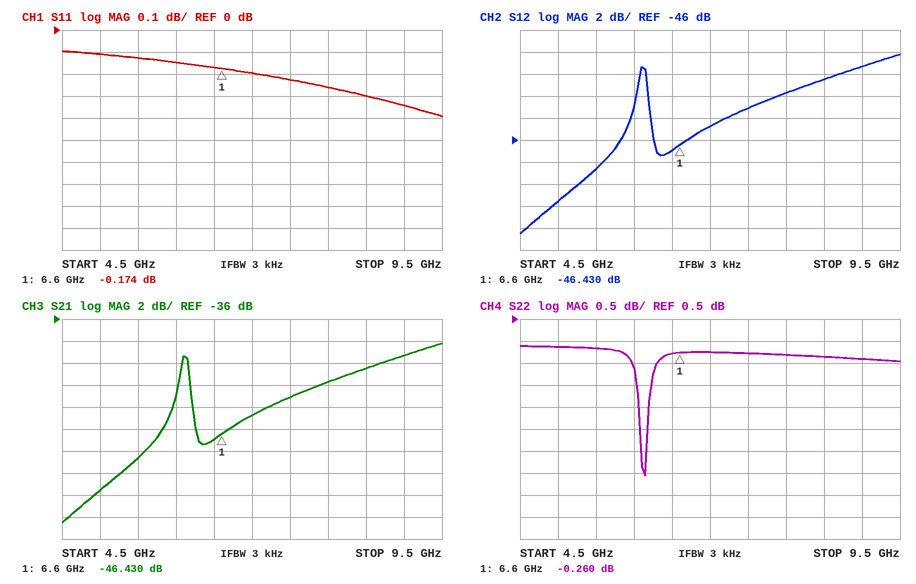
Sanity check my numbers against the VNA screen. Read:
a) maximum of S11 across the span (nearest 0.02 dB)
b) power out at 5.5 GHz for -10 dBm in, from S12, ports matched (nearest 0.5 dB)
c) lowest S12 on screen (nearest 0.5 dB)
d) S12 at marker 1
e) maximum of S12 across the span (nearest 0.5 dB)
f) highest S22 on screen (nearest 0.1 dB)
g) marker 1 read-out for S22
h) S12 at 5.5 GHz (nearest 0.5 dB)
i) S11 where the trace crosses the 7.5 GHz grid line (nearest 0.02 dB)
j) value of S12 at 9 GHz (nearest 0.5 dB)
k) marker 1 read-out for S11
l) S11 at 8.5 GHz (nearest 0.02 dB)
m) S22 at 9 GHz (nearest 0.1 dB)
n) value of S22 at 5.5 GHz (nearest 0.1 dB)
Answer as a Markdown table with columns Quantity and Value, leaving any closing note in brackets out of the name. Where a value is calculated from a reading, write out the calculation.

| Quantity | Value |
|---|---|
| maximum of S11 across the span | -0.10 dB |
| power out at 5.5 GHz for -10 dBm in, from S12, ports matched | -10 dBm + (-48.5 dB) = -58.5 dBm |
| lowest S12 on screen | -54.5 dB |
| S12 at marker 1 | -46.430 dB |
| maximum of S12 across the span | -38.0 dB |
| highest S22 on screen | -0.1 dB |
| marker 1 read-out for S22 | -0.260 dB |
| S12 at 5.5 GHz | -48.5 dB |
| S11 where the trace crosses the 7.5 GHz grid line | -0.22 dB |
| value of S12 at 9 GHz | -39.5 dB |
| marker 1 read-out for S11 | -0.174 dB |
| S11 at 8.5 GHz | -0.30 dB |
| S22 at 9 GHz | -0.4 dB |
| value of S22 at 5.5 GHz | -0.2 dB |
